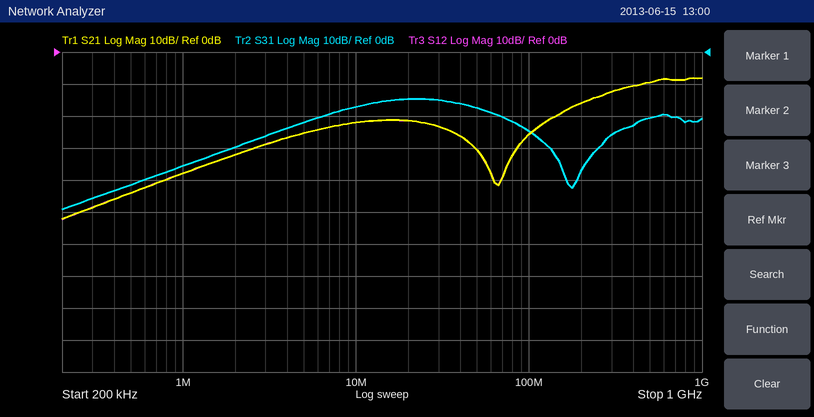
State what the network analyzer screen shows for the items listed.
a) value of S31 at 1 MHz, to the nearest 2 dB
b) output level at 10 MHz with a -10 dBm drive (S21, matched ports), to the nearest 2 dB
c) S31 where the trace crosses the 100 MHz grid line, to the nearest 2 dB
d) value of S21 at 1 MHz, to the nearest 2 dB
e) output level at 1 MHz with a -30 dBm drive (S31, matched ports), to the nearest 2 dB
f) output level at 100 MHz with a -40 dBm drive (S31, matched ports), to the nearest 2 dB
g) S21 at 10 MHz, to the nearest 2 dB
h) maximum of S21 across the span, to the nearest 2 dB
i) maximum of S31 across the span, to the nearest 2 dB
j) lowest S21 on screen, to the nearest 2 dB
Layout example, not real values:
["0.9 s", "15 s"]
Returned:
["-36 dB", "-32 dBm", "-24 dB", "-38 dB", "-66 dBm", "-64 dBm", "-22 dB", "-8 dB", "-14 dB", "-52 dB"]
